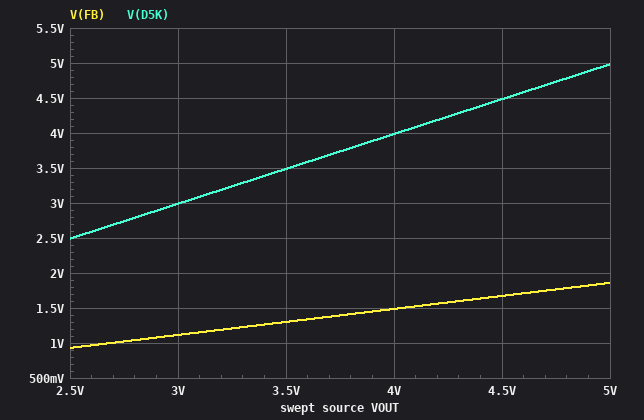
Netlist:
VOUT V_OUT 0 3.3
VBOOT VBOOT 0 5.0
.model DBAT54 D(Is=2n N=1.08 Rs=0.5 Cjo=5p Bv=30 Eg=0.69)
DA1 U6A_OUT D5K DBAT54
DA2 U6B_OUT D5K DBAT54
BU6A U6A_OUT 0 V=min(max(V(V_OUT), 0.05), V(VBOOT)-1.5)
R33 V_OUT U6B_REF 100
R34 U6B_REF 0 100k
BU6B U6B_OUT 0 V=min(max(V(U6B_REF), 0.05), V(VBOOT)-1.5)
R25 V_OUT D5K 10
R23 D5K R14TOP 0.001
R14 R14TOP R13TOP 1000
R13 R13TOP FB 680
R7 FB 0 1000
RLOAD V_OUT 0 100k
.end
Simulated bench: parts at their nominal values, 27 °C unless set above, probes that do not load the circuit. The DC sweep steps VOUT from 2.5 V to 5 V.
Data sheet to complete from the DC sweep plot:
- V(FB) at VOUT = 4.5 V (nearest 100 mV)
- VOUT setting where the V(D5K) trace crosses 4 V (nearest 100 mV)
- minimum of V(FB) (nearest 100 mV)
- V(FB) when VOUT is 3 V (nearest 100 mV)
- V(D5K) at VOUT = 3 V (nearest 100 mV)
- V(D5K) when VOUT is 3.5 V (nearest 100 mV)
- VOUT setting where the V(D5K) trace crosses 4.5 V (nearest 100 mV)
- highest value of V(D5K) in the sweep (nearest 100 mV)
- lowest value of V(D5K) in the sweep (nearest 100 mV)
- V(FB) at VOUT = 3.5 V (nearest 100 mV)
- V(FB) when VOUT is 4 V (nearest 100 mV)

1.7 V
4.0 V
900 mV
1.1 V
3.0 V
3.5 V
4.5 V
5.0 V
2.5 V
1.3 V
1.5 V
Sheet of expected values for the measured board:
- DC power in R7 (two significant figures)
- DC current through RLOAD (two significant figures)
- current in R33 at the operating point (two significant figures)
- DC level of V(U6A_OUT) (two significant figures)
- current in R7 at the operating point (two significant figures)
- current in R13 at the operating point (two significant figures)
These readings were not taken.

1.5 mW
33 µA
33 µA
3.3 V
1.2 mA
1.2 mA
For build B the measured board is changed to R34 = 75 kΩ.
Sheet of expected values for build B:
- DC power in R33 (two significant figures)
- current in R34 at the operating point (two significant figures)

190 nW
44 µA
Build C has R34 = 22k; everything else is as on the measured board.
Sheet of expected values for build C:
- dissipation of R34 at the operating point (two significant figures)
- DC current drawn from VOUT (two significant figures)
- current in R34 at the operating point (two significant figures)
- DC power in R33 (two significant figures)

490 µW
1.4 mA
150 µA
2.2 µW
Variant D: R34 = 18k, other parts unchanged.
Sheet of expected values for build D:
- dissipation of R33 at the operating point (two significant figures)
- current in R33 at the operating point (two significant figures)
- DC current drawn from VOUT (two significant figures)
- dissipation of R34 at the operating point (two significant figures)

3.3 µW
180 µA
1.4 mA
600 µW
